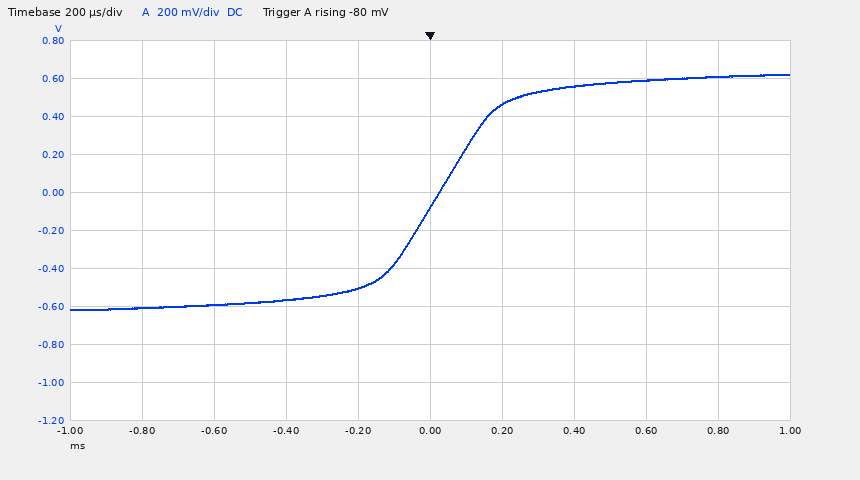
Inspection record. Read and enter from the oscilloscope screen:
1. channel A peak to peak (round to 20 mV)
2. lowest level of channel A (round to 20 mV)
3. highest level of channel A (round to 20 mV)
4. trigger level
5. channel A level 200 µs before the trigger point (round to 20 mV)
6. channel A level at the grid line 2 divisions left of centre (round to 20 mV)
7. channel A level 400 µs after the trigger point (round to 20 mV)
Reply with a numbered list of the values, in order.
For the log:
1. 1.24 V
2. -620 mV
3. 620 mV
4. -80 mV
5. -500 mV
6. -560 mV
7. 560 mV
